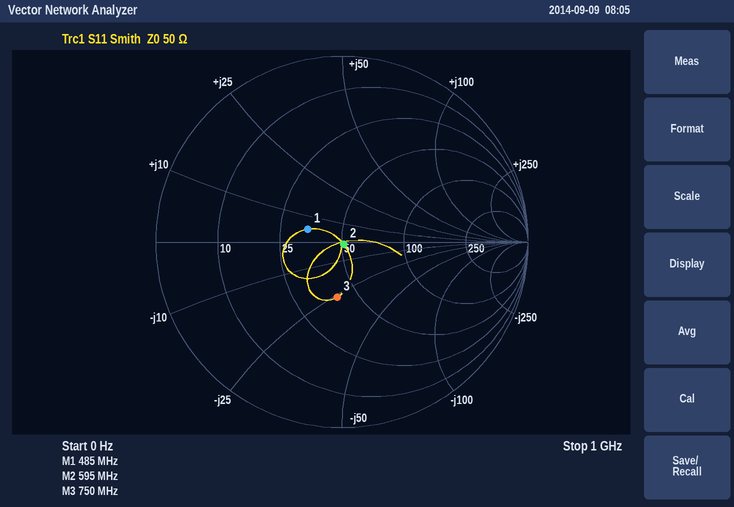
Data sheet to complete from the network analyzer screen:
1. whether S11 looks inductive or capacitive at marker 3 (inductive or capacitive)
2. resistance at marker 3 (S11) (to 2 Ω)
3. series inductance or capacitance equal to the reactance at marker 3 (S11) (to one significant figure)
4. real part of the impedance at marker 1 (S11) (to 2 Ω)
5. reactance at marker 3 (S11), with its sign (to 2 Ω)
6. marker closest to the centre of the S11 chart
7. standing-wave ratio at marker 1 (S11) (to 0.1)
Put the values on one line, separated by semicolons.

capacitive; 40 Ω; 8 pF; 34 Ω; -26 Ω; marker 2; 1.5
